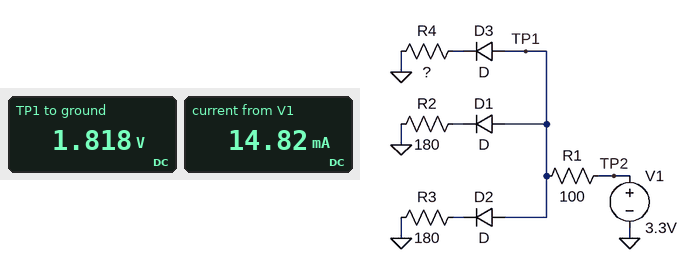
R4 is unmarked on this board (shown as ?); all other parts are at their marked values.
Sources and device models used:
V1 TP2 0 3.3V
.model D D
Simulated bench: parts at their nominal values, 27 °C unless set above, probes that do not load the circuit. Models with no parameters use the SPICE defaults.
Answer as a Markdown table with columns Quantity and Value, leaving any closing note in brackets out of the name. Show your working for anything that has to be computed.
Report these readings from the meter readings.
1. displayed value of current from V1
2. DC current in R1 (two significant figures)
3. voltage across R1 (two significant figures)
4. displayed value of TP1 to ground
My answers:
| Quantity | Value |
|---|---|
| displayed value of current from V1 | 14.82 mA |
| DC current in R1 | (3.3 V - 1.818 V) / 100 Ω = 15 mA |
| voltage across R1 | 3.3 V - 1.818 V = 1.5 V |
| displayed value of TP1 to ground | 1.818 V |
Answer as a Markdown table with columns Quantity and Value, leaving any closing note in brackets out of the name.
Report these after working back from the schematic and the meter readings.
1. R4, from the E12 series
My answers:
| Quantity | Value |
|---|---|
| R4, from the E12 series | 470 Ω |
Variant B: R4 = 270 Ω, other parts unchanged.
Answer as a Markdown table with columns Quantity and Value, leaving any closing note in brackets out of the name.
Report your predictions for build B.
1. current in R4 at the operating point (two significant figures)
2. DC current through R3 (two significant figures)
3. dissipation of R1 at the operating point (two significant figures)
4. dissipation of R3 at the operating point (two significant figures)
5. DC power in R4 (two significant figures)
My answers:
| Quantity | Value |
|---|---|
| current in R4 at the operating point | 3.9 mA |
| DC current through R3 | 5.8 mA |
| dissipation of R1 at the operating point | 24 mW |
| dissipation of R3 at the operating point | 6.1 mW |
| DC power in R4 | 4.1 mW |
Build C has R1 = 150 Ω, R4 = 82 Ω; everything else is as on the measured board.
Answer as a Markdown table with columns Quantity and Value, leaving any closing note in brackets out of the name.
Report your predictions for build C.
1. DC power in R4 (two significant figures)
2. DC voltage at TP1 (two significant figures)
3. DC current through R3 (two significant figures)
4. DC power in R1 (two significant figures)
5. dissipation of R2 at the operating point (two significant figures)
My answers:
| Quantity | Value |
|---|---|
| DC power in R4 | 4.0 mW |
| DC voltage at TP1 | 1.3 V |
| DC current through R3 | 3.3 mA |
| DC power in R1 | 27 mW |
| dissipation of R2 at the operating point | 1.9 mW |
